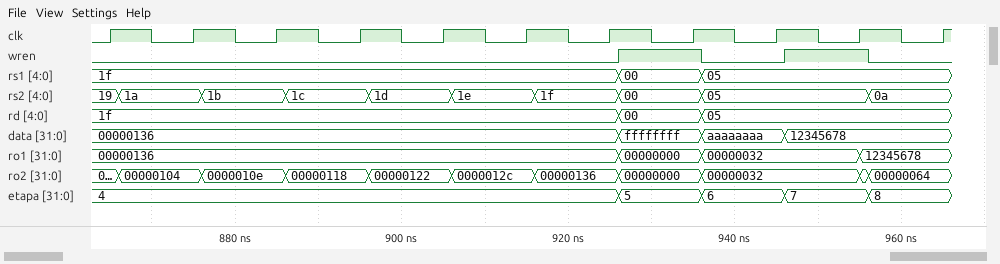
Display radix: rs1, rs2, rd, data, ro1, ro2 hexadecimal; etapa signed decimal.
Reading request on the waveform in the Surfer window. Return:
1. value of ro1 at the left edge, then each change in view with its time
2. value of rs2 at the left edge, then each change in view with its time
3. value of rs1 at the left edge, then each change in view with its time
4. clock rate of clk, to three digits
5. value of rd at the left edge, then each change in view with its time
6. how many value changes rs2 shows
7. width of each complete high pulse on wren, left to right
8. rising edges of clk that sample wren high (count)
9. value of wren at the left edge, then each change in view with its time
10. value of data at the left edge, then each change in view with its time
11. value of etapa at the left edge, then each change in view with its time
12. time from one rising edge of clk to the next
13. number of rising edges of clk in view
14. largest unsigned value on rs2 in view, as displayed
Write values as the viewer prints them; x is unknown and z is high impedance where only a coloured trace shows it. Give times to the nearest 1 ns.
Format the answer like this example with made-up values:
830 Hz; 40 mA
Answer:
00000136, 00000000 at 926 ns, 00000032 at 936 ns, 12345678 at 955 ns; 19, 1a at 866 ns, 1b at 876 ns, 1c at 886 ns, 1d at 896 ns, 1e at 906 ns, 1f at 916 ns, 00 at 926 ns, 05 at 936 ns, 0a at 956 ns; 1f, 00 at 926 ns, 05 at 936 ns; 100 MHz; 1f, 00 at 926 ns, 05 at 936 ns; 9; 10 ns, 10 ns; 2; 0, 1 at 926 ns, 0 at 936 ns, 1 at 946 ns, 0 at 956 ns; 00000136, ffffffff at 926 ns, aaaaaaaa at 936 ns, 12345678 at 946 ns; 4, 5 at 926 ns, 6 at 936 ns, 7 at 946 ns, 8 at 956 ns; 10 ns; 11; 1f
